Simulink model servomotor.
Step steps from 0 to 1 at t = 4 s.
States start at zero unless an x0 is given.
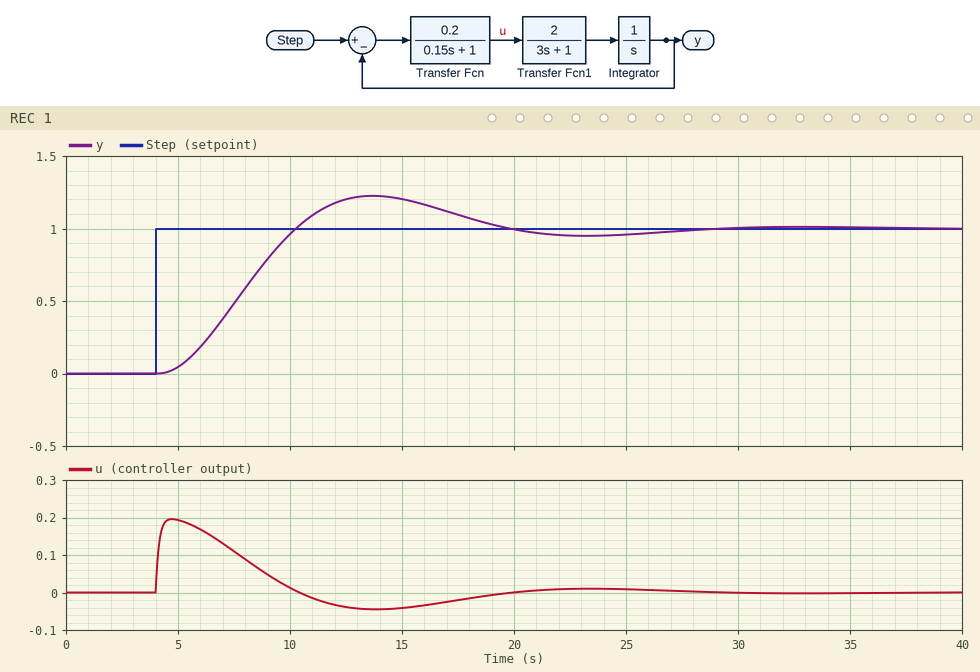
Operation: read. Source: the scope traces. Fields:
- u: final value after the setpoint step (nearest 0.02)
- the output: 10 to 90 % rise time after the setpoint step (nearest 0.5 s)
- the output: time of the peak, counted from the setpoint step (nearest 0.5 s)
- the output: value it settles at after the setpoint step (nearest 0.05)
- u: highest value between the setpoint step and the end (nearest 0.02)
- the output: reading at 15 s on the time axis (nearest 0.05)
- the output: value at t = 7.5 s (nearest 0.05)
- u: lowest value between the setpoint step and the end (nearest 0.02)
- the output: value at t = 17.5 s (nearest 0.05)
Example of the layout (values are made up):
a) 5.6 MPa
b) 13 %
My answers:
a) 0.00
b) 4.0 s
c) 9.5 s
d) 1.00
e) 0.20
f) 1.20
g) 0.50
h) -0.04
i) 1.10
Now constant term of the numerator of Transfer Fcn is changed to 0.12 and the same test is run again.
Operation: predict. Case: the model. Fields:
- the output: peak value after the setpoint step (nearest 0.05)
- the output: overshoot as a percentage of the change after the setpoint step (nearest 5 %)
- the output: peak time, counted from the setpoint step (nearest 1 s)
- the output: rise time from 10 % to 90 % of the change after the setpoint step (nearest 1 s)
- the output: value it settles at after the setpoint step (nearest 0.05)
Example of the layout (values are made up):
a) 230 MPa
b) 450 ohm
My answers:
a) 1.10
b) 10 %
c) 14 s
d) 6 s
e) 1.00
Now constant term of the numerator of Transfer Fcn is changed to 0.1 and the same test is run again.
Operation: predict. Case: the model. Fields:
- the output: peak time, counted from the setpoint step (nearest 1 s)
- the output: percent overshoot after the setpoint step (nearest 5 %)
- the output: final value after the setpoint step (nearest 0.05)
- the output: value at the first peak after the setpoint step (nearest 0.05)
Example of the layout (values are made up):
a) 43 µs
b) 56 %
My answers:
a) 16 s
b) 10 %
c) 1.00
d) 1.10
